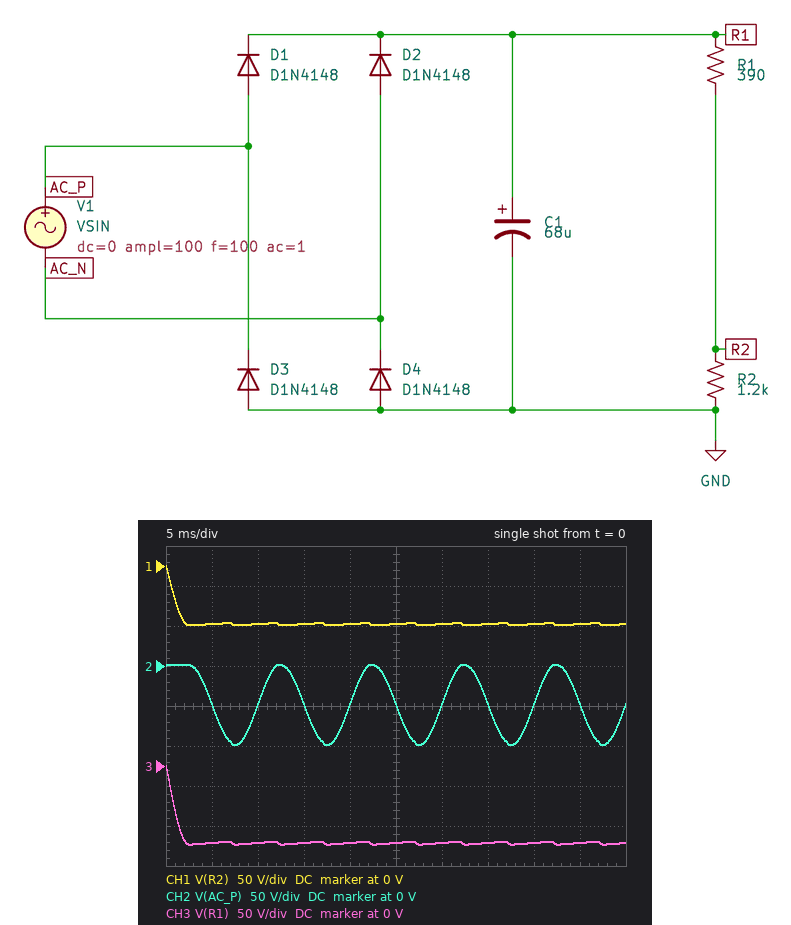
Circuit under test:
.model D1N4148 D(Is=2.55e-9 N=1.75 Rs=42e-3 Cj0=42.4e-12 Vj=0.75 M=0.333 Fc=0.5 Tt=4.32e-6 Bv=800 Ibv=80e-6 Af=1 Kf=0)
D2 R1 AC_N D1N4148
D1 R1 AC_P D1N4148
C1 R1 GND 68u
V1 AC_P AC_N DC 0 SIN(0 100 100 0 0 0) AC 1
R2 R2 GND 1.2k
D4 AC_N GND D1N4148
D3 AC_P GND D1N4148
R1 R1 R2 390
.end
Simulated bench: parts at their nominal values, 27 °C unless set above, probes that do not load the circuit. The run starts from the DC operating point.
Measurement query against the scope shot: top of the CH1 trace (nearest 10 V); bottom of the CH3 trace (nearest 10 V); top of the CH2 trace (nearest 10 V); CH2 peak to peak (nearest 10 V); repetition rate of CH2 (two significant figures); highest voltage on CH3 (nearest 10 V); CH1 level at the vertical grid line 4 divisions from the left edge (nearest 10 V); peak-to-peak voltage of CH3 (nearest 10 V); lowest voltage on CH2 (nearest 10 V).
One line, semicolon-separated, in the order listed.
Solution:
0 V; -100 V; 0 V; 100 V; 100 Hz; 0 V; -70 V; 100 V; -100 V
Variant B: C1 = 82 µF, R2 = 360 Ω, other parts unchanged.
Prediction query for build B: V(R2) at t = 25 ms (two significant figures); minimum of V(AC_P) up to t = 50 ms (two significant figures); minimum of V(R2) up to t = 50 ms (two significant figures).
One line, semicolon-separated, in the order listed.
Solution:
-45 V; -99 V; -47 V
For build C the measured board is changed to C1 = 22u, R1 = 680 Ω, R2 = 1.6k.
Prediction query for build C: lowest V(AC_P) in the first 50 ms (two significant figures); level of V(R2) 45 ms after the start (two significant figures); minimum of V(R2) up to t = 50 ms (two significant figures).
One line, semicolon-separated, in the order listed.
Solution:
-99 V; -66 V; -69 V
